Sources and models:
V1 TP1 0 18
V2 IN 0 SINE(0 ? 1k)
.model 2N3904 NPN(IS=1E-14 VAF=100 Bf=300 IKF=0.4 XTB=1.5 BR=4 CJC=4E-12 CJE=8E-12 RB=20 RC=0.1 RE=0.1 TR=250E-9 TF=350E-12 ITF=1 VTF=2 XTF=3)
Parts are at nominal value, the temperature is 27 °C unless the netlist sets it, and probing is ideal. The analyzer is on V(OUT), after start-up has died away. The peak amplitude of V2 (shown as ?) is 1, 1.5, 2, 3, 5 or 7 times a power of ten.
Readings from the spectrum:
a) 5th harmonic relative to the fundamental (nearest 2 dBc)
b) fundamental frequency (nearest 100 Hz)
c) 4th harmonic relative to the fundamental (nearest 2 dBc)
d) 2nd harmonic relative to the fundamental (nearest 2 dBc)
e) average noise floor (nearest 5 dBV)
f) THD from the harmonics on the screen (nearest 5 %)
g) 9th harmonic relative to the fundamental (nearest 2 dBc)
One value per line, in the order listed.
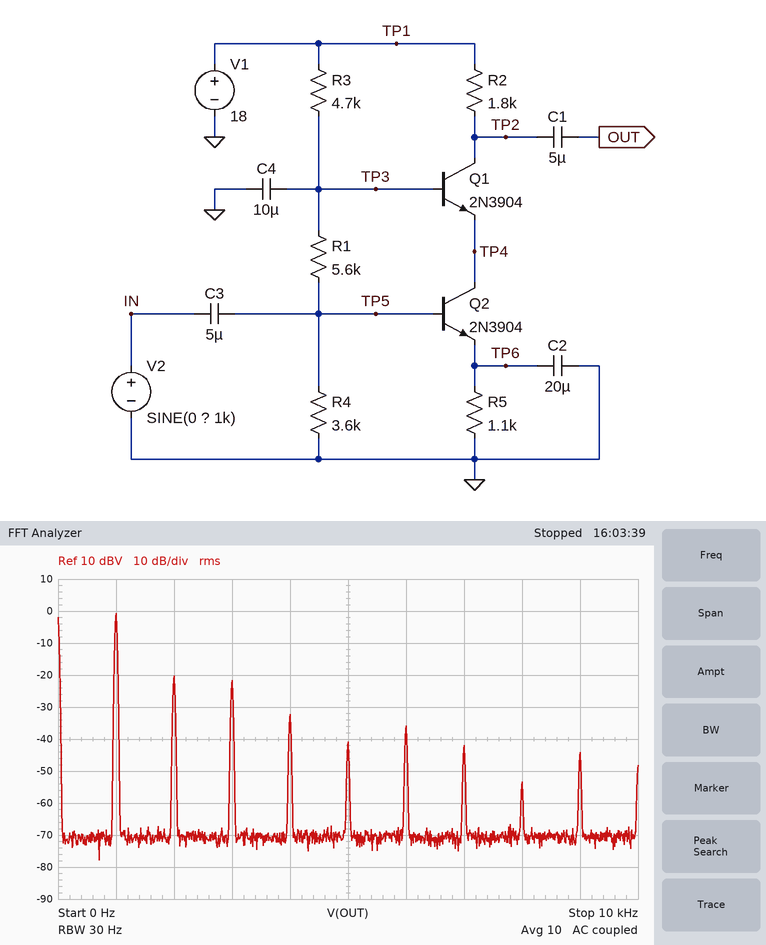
-40 dBc
1.0 kHz
-32 dBc
-20 dBc
-70 dBV
15 %
-44 dBc
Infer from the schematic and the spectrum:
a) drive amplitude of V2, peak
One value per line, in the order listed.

10 mV
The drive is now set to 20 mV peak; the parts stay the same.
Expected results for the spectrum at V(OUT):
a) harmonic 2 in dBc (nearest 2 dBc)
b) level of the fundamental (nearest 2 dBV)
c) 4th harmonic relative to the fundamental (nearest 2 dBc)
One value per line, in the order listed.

-22 dBc
4 dBV
-30 dBc
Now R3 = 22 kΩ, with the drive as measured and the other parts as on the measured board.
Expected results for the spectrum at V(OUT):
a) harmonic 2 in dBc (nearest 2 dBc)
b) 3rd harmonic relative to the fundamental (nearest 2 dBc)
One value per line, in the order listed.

-22 dBc
-46 dBc
